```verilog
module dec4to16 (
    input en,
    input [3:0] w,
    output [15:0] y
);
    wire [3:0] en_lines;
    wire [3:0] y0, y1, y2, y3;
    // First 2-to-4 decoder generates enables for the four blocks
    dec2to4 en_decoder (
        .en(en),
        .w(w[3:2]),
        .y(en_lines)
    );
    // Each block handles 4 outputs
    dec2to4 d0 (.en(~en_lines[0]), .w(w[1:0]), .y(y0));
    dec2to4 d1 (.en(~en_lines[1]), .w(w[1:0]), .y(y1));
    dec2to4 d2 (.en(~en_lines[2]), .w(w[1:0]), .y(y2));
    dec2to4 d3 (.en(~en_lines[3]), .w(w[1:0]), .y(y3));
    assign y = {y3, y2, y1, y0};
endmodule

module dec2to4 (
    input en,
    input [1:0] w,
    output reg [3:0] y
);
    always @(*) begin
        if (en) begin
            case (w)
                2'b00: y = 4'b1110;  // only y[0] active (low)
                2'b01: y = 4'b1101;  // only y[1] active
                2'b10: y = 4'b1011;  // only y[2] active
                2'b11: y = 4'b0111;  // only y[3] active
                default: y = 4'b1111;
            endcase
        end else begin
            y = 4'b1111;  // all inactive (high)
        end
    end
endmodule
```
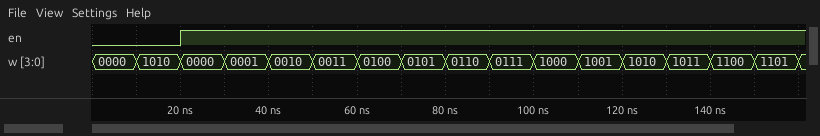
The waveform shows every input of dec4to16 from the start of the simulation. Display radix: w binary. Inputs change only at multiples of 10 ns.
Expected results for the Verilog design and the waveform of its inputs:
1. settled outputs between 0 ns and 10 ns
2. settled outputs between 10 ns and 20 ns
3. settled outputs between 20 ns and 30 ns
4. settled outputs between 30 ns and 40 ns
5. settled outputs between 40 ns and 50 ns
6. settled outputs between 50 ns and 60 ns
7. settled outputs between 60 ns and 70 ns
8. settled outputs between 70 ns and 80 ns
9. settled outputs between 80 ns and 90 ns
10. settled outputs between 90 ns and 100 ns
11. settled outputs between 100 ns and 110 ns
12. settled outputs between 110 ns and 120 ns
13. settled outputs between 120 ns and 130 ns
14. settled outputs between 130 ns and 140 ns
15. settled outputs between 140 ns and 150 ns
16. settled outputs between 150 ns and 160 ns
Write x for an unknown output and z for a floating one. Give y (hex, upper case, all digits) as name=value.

y=FFFF
y=FFFF
y=FFFE
y=FFFD
y=FFFB
y=FFF7
y=FFEF
y=FFDF
y=FFBF
y=FF7F
y=FEFF
y=FDFF
y=FBFF
y=F7FF
y=EFFF
y=DFFF
